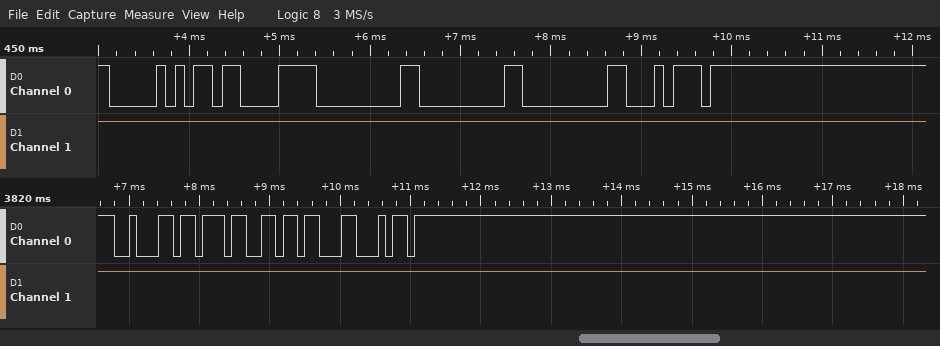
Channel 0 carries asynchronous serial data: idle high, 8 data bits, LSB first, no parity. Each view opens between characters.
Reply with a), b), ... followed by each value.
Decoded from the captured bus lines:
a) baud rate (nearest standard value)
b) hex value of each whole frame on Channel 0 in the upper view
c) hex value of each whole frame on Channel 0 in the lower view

a) 9600 baud
b) 50, C3, 00, 00, 00, 74
c) 62, 37, 1B, B4
